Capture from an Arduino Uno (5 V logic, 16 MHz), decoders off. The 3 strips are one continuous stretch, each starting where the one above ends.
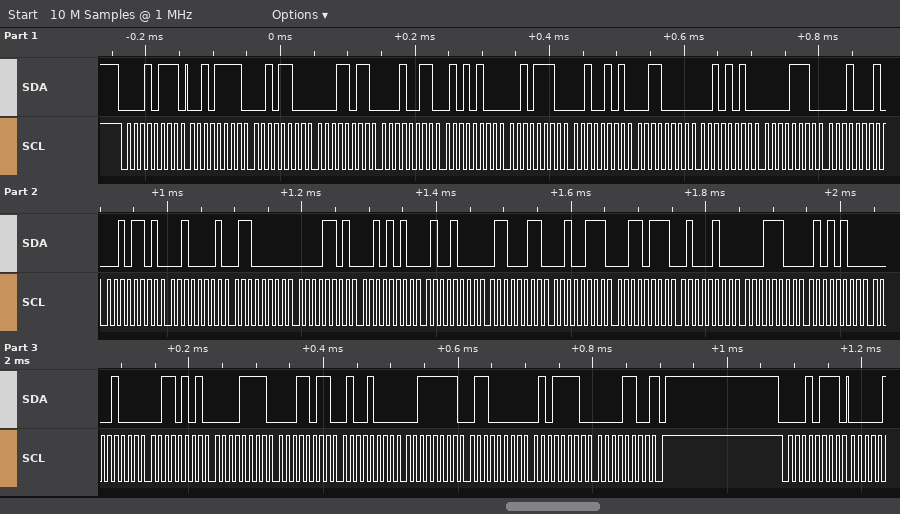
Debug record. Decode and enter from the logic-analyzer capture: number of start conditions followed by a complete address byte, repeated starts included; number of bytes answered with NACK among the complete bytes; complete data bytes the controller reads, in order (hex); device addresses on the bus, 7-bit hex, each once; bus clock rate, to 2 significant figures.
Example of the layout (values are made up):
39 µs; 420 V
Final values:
2; 1; 2F 2C 1B 13 54 2E 25 30 2A 0E 11 2D 21 60 0D 2A 48 63 27 37 44 1C 54 08 35 0F 1B 48 3F 60 5E 0C; 0x0B; 100 kHz
